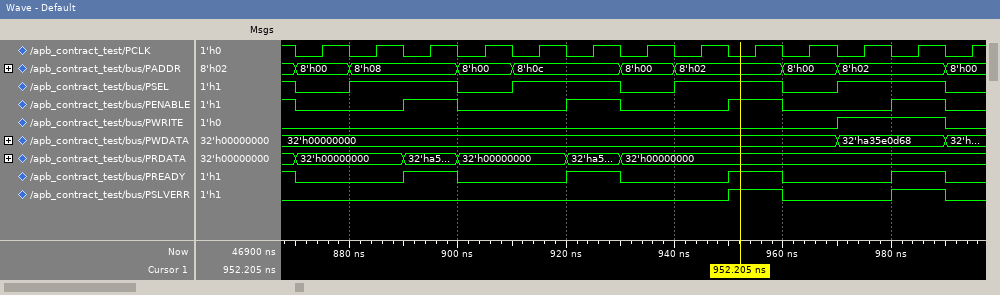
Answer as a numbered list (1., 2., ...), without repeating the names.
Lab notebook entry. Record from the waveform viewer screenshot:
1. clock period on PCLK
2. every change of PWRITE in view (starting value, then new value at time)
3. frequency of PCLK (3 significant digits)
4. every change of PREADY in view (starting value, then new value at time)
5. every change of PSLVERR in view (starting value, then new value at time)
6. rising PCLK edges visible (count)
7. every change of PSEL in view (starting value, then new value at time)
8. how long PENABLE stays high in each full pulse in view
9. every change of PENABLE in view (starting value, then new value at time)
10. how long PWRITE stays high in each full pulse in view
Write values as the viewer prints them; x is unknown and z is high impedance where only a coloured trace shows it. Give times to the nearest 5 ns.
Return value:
1. 10 ns
2. 0, 1 at 970 ns, 0 at 990 ns
3. 100 MHz
4. 1, 0 at 870 ns, 1 at 890 ns, 0 at 900 ns, 1 at 920 ns, 0 at 930 ns, 1 at 950 ns, 0 at 960 ns, 1 at 980 ns, 0 at 990 ns
5. 0, 1 at 950 ns, 0 at 960 ns, 1 at 980 ns, 0 at 990 ns
6. 13
7. 1, 0 at 870 ns, 1 at 880 ns, 0 at 900 ns, 1 at 910 ns, 0 at 930 ns, 1 at 940 ns, 0 at 960 ns, 1 at 970 ns, 0 at 990 ns
8. 10 ns, 10 ns, 10 ns, 10 ns
9. 1, 0 at 870 ns, 1 at 890 ns, 0 at 900 ns, 1 at 920 ns, 0 at 930 ns, 1 at 950 ns, 0 at 960 ns, 1 at 980 ns, 0 at 990 ns
10. 20 ns
